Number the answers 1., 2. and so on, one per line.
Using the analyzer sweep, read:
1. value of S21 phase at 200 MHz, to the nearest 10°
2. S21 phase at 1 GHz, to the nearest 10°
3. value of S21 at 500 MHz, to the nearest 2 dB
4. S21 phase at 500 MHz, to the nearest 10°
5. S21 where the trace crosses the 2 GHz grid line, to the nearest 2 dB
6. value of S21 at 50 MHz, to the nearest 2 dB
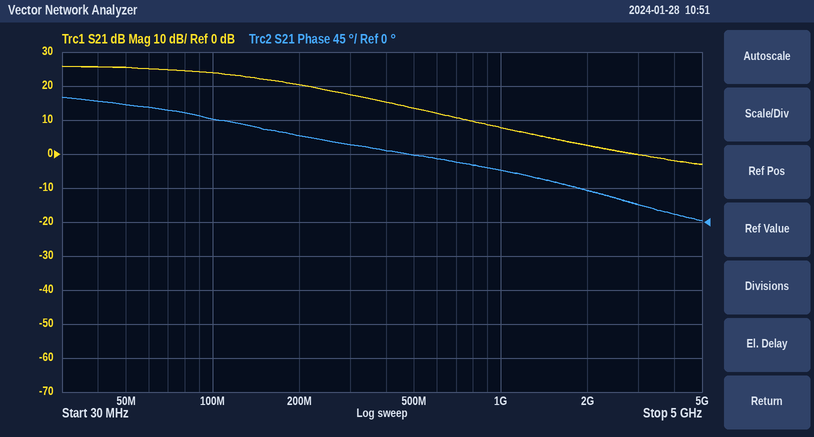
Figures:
1. 110°
2. 70°
3. 14 dB
4. 90°
5. 2 dB
6. 26 dB
